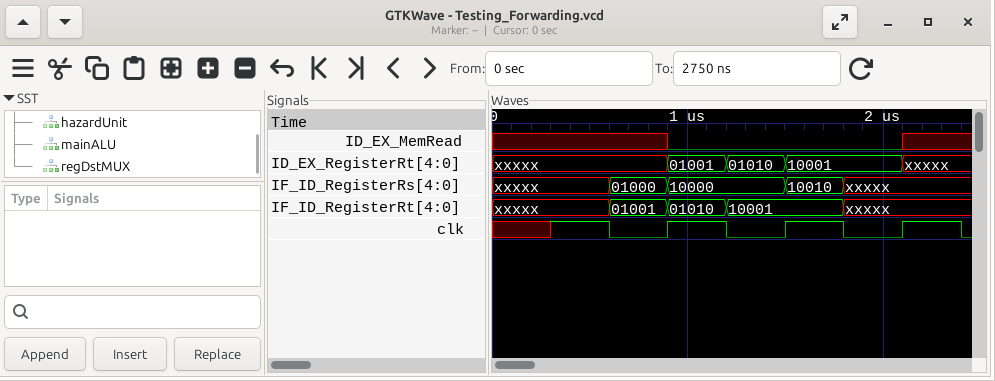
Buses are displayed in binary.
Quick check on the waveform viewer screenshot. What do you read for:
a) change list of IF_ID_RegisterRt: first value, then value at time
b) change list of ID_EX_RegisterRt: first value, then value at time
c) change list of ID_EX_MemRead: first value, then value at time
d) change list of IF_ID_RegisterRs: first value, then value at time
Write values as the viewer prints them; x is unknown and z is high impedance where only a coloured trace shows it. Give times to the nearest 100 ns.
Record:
xxxxx, 01001 at 600 ns, 01010 at 900 ns, 10001 at 1200 ns, xxxxx at 1800 ns
xxxxx, 01001 at 900 ns, 01010 at 1200 ns, 10001 at 1500 ns, xxxxx at 2100 ns
x, 0 at 900 ns, x at 2100 ns
xxxxx, 01000 at 600 ns, 10000 at 900 ns, 10010 at 1500 ns, xxxxx at 1800 ns
